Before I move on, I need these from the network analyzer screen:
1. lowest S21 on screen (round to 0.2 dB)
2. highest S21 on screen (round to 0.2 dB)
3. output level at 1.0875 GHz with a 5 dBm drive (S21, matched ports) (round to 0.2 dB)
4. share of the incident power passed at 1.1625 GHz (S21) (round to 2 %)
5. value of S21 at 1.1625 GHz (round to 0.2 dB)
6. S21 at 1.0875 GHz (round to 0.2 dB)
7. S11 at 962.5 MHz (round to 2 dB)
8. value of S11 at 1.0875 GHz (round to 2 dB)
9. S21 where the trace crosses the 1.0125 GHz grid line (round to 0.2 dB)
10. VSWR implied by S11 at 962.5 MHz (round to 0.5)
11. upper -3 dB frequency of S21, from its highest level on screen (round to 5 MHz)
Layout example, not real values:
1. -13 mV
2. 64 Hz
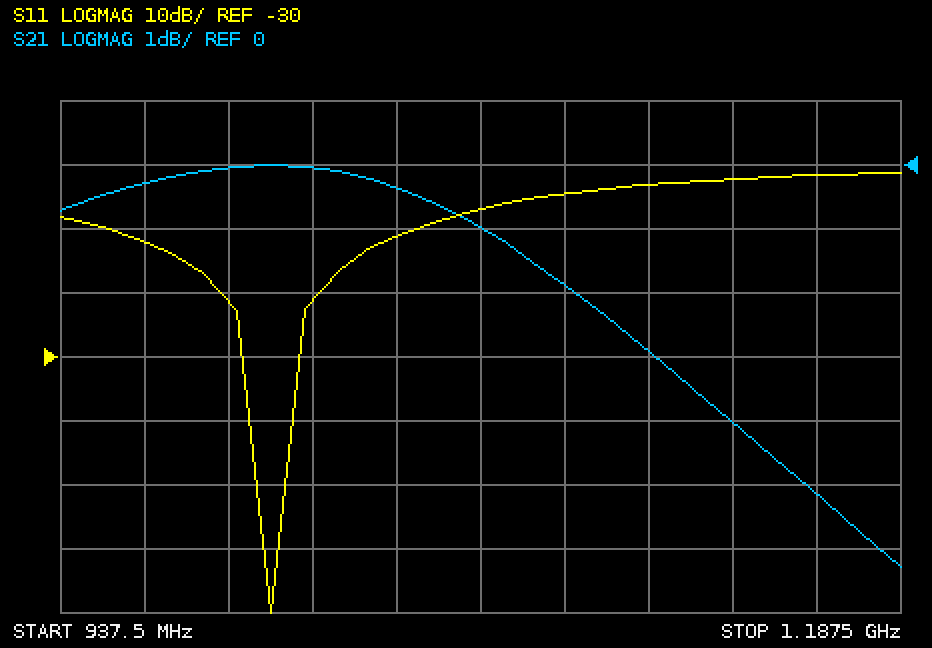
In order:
1. -6.2 dB
2. 0.0 dB
3. 3.2 dBm
4. 30 %
5. -5.2 dB
6. -1.8 dB
7. -12 dB
8. -4 dB
9. 0.0 dB
10. 1.5
11. 1.115 GHz
